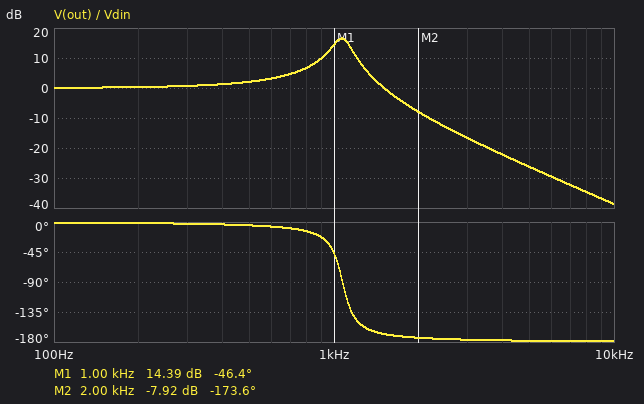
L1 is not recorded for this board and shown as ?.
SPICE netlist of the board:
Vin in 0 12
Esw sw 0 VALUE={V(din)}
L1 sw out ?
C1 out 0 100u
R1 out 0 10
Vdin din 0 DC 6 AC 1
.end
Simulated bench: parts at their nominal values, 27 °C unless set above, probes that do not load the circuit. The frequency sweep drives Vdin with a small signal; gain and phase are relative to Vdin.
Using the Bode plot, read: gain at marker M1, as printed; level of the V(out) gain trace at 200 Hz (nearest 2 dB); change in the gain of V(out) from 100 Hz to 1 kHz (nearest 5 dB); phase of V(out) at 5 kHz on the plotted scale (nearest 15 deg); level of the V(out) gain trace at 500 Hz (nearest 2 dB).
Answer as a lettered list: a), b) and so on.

a) 14.39 dB
b) 0 dB
c) 15 dB
d) -180 deg
e) 2 dB
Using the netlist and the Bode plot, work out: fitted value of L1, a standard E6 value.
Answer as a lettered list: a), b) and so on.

a) 220 µH
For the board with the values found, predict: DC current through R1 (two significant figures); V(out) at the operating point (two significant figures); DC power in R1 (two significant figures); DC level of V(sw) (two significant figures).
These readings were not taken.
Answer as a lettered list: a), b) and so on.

a) 600 mA
b) 6.0 V
c) 3.6 W
d) 6.0 V
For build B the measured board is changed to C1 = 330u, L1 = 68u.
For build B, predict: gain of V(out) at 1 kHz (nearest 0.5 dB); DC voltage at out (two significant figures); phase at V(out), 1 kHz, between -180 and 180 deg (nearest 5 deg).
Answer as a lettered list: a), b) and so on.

a) 18.5 dB
b) 6.0 V
c) -20 deg
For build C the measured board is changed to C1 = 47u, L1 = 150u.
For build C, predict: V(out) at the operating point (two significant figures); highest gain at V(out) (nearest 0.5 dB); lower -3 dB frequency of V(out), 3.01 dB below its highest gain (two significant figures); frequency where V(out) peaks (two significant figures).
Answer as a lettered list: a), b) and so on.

a) 6.0 V
b) 15.0 dB
c) 1.7 kHz
d) 1.9 kHz
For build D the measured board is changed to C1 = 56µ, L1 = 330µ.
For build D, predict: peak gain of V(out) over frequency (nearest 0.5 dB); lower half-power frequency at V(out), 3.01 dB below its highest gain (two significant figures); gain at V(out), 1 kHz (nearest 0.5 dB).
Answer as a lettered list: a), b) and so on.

a) 12.5 dB
b) 1.0 kHz
c) 9.5 dB
